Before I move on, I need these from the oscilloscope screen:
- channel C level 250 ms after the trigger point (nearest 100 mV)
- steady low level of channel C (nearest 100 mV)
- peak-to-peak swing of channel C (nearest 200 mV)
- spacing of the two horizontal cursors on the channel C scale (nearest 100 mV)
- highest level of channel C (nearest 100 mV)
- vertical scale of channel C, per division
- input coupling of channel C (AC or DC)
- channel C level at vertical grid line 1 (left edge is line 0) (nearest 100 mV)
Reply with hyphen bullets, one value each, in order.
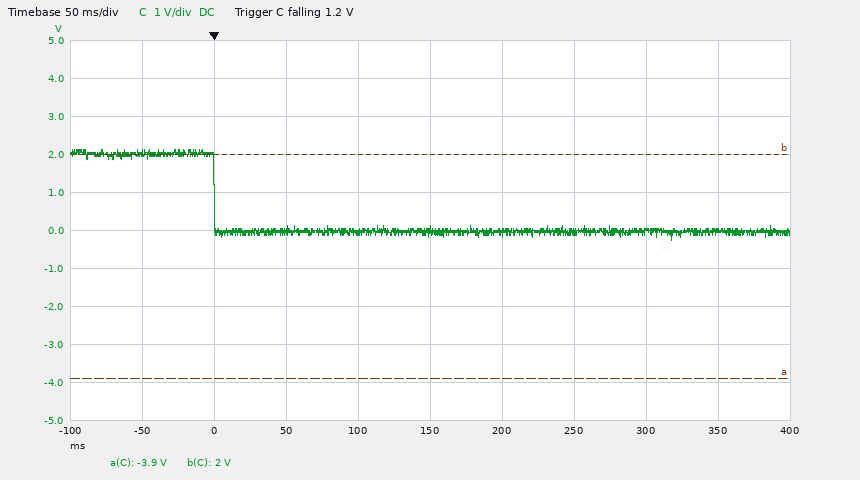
- 0.0 V
- 0.0 V
- 2.4 V
- 5.9 V
- 2.1 V
- 1 V
- DC
- 2.0 V
